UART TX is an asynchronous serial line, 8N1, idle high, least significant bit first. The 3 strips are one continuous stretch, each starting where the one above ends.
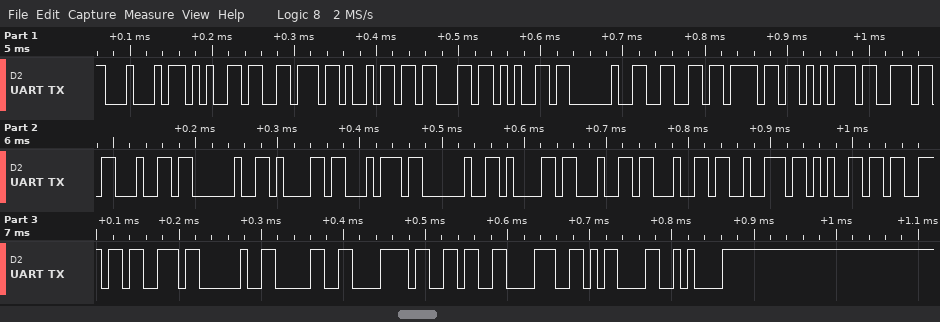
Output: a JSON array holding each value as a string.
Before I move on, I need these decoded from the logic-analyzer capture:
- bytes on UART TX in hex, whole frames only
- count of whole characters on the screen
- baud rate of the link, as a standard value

["0x44 0x65 0x76 0x69 0x63 0x65 0x20 0x66 0x6F 0x75 0x6E 0x64 0x20 0x61 0x74 0x20 0x61 0x64 0x64 0x72 0x65 0x73 0x73 0x20 0x30 0x78 0x36 0x38 0x0D 0x0A", "30", "115200 baud"]
